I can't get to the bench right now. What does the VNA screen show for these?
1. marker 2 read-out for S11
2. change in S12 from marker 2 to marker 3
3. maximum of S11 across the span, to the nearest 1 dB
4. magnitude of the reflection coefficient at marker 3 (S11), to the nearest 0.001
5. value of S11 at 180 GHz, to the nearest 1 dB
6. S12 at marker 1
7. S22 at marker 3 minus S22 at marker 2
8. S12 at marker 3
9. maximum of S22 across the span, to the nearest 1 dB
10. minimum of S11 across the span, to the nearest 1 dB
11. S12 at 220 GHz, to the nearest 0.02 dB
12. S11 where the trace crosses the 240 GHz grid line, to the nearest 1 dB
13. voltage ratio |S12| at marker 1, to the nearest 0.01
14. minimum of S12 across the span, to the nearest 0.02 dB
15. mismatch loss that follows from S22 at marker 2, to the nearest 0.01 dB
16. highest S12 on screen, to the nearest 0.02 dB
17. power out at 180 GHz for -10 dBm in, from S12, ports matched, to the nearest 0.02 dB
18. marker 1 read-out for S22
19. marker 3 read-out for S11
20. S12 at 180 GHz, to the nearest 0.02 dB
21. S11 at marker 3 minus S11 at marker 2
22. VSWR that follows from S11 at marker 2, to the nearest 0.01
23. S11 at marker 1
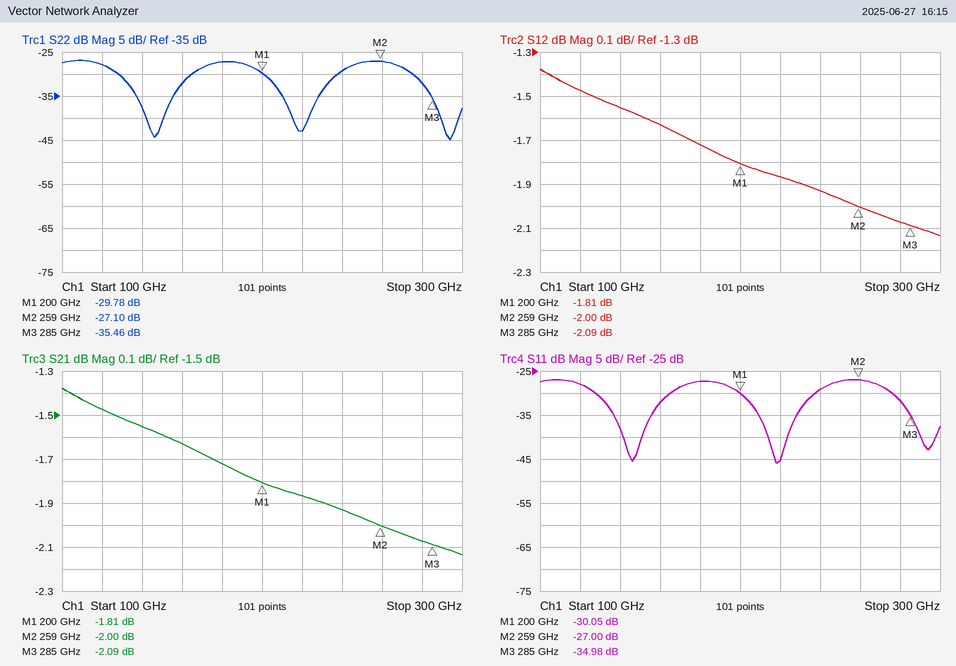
-27.00 dB
-0.09 dB
-27 dB
0.018
-27 dB
-1.81 dB
-8.36 dB
-2.09 dB
-27 dB
-46 dB
-1.86 dB
-29 dB
0.81
-2.14 dB
0.01 dB
-1.38 dB
-11.72 dBm
-29.78 dB
-34.98 dB
-1.72 dB
-7.98 dB
1.09
-30.05 dB
